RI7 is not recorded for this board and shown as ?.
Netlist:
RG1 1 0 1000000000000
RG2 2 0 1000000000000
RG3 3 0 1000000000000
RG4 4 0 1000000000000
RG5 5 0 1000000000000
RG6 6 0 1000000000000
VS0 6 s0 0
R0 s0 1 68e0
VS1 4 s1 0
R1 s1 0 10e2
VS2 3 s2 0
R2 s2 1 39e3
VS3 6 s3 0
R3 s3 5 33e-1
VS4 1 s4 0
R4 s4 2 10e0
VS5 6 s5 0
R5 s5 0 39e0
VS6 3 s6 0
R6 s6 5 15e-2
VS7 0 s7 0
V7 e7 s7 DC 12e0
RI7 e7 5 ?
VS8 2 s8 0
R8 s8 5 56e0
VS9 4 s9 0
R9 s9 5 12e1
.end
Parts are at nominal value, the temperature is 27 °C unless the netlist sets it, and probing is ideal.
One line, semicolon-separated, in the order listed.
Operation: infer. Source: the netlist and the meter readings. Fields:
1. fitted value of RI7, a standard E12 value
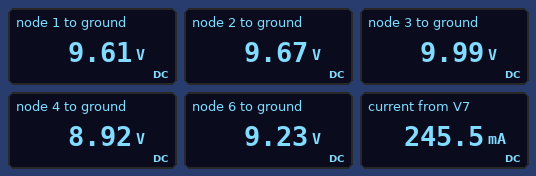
8.2 Ω
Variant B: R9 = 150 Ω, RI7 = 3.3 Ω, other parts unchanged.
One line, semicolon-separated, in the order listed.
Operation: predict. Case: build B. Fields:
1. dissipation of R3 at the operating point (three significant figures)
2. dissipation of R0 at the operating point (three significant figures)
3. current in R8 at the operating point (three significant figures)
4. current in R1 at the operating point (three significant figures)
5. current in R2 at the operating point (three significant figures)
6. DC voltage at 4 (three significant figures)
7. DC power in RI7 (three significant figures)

217 mW; 2.72 mW; 6.31 mA; 9.65 mA; 10.7 µA; 9.65 V; 245 mW
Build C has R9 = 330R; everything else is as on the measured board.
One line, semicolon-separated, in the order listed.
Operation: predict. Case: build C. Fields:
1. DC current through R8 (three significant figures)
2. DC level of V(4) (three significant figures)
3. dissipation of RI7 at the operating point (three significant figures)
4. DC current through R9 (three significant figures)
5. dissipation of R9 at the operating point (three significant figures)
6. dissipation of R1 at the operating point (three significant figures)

5.69 mA; 7.52 V; 489 mW; 7.52 mA; 18.6 mW; 56.5 mW
